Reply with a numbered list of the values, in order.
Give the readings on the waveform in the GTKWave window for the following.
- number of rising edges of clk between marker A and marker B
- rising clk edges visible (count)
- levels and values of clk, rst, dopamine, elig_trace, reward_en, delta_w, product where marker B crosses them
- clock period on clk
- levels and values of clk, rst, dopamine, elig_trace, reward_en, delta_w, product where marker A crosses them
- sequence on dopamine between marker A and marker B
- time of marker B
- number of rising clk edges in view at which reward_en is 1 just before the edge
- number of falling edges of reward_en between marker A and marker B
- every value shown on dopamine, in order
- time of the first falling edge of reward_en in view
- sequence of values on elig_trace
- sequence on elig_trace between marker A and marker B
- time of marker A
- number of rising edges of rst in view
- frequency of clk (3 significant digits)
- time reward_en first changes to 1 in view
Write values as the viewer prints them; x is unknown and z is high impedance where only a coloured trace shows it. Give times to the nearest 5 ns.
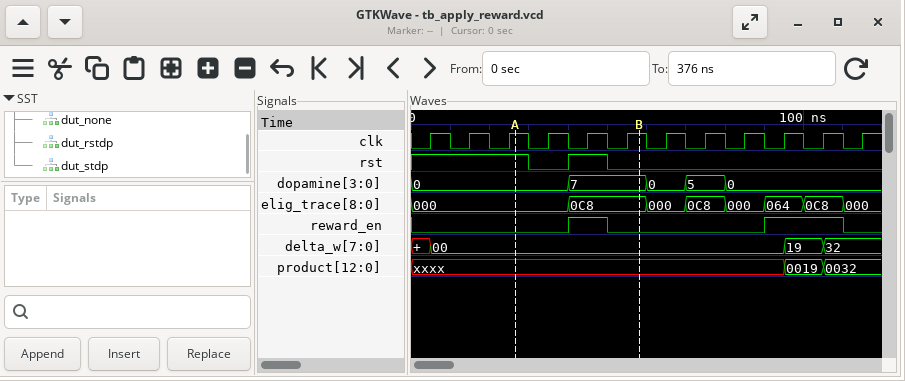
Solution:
1. 3
2. 12
3. clk=1, rst=0, dopamine=7, elig_trace=0C8, reward_en=0, delta_w=00, product=xxxx
4. 10 ns
5. clk=1, rst=1, dopamine=0, elig_trace=000, reward_en=0, delta_w=00, product=xxxx
6. 0, 7
7. 60 ns
8. 3
9. 1
10. 0, 7, 0, 5, 0
11. 50 ns
12. 000, 0C8, 000, 0C8, 000, 064, 0C8, 000
13. 000, 0C8
14. 25 ns
15. 1
16. 100 MHz
17. 40 ns
